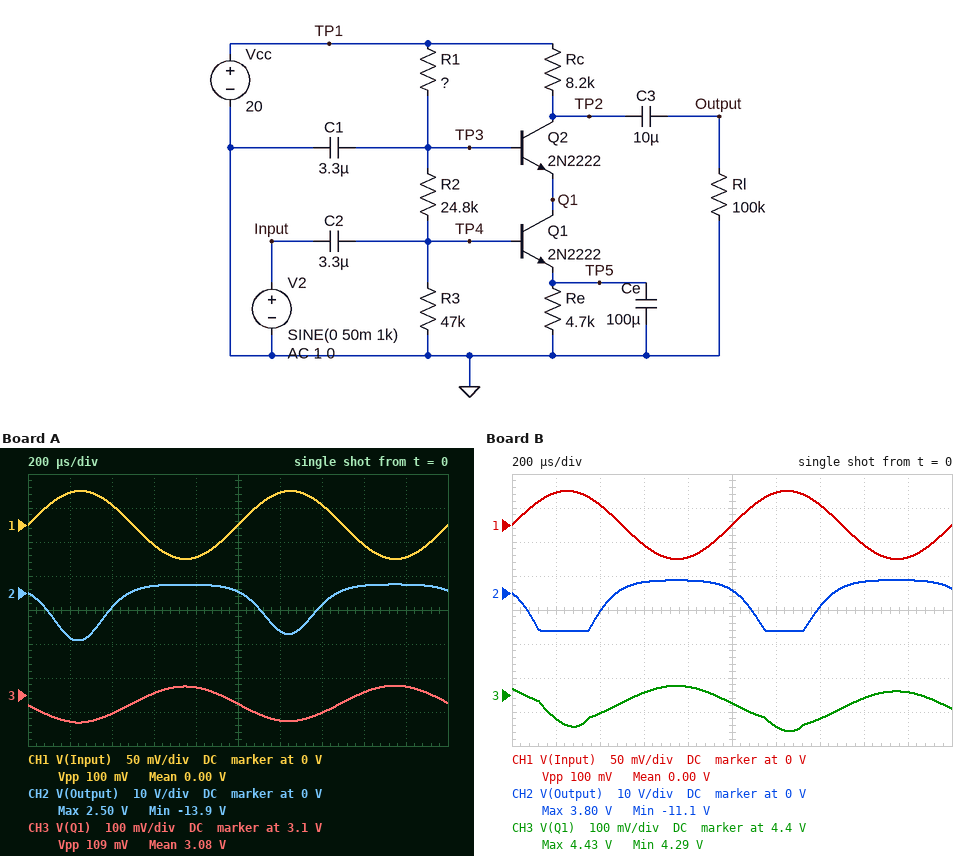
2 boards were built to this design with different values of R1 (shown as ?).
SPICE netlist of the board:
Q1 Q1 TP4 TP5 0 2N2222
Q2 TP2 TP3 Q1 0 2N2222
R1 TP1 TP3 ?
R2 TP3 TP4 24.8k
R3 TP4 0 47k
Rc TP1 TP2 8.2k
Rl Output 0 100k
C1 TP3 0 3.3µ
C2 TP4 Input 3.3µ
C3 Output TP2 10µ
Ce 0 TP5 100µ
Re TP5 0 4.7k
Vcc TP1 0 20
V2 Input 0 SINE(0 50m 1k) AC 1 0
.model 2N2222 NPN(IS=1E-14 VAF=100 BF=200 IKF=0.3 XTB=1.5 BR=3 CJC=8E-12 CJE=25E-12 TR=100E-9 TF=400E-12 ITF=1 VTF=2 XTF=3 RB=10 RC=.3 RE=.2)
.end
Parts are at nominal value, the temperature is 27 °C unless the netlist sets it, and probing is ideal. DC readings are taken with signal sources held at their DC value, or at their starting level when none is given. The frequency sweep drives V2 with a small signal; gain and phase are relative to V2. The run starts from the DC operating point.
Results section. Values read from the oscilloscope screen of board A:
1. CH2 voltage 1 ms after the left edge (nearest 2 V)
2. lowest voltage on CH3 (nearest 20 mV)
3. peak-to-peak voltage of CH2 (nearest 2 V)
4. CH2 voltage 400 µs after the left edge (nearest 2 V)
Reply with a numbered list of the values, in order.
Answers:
1. 0 V
2. 3.02 V
3. 16 V
4. -4 V
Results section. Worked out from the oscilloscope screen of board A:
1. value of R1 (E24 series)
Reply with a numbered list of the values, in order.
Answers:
1. 300 kΩ
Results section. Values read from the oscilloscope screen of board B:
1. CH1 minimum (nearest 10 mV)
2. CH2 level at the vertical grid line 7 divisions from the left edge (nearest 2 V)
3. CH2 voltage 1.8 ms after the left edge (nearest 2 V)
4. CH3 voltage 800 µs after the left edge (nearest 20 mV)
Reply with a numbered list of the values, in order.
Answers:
1. -50 mV
2. -4 V
3. 4 V
4. 4.42 V
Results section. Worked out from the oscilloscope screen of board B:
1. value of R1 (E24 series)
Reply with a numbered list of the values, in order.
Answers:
1. 200 kΩ
